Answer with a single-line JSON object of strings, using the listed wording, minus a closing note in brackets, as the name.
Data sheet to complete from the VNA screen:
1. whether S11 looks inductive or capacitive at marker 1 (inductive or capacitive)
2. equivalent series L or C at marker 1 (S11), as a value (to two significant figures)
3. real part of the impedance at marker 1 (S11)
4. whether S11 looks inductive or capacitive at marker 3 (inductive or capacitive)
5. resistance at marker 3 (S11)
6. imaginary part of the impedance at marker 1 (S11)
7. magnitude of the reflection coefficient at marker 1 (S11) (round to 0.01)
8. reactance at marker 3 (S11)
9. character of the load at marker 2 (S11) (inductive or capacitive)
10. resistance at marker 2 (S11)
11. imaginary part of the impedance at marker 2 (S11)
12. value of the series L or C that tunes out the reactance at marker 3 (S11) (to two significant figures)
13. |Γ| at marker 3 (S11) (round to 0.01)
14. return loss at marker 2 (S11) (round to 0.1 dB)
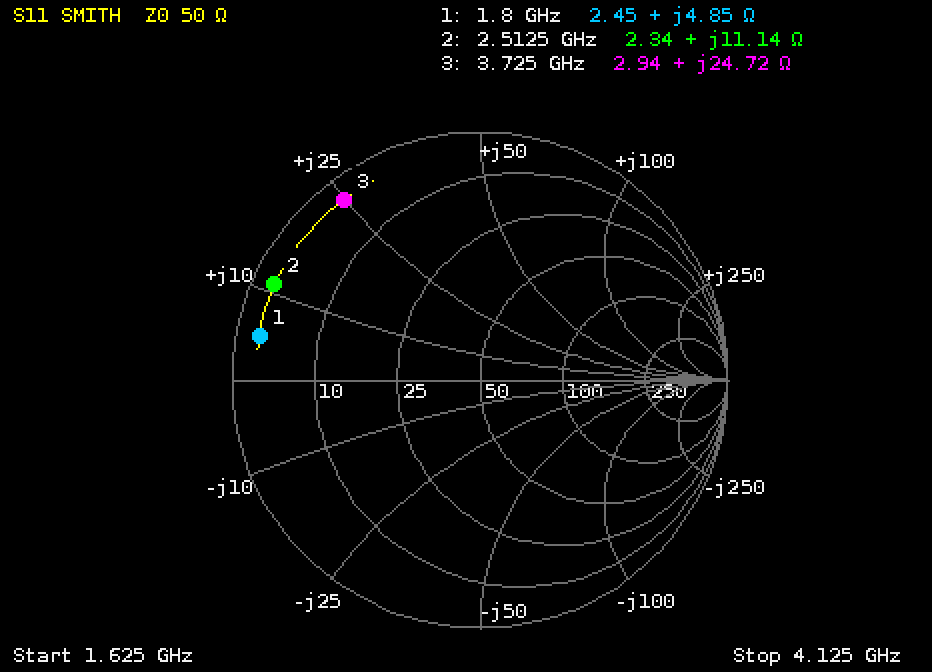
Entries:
{"whether S11 looks inductive or capacitive at marker 1": "inductive", "equivalent series L or C at marker 1 (S11), as a value": "430 pH", "real part of the impedance at marker 1": "2.45 Ω", "whether S11 looks inductive or capacitive at marker 3": "inductive", "resistance at marker 3": "2.94 Ω", "imaginary part of the impedance at marker 1": "+4.85 Ω", "magnitude of the reflection coefficient at marker 1 (S11)": "0.91", "reactance at marker 3": "+24.72 Ω", "character of the load at marker 2 (S11)": "inductive", "resistance at marker 2": "2.34 Ω", "imaginary part of the impedance at marker 2": "+11.14 Ω", "value of the series L or C that tunes out the reactance at marker 3 (S11)": "1.7 pF", "|Γ| at marker 3 (S11)": "0.91", "return loss at marker 2 (S11)": "0.8 dB"}
